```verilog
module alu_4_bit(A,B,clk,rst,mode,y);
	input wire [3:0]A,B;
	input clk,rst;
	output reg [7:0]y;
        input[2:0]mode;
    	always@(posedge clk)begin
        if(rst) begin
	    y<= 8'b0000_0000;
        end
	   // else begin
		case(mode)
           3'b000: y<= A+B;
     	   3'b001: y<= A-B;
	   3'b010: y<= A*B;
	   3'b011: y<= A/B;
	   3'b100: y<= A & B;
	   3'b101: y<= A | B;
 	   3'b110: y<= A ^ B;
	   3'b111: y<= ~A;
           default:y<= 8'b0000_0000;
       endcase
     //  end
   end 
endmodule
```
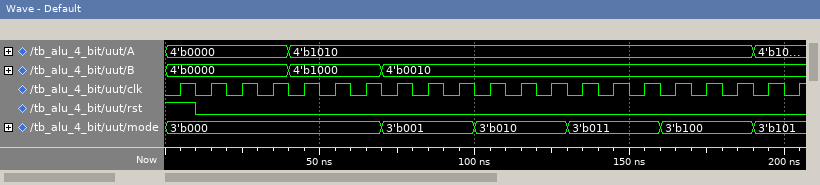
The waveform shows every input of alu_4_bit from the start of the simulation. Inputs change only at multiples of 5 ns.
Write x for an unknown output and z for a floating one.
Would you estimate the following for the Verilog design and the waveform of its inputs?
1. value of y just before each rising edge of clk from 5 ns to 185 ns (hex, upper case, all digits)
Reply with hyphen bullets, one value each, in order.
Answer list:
- x, 00, 00, 00, 00, 12, 12, 12, 08, 08, 08, 14, 14, 14, 05, 05, 05, 02, 02
